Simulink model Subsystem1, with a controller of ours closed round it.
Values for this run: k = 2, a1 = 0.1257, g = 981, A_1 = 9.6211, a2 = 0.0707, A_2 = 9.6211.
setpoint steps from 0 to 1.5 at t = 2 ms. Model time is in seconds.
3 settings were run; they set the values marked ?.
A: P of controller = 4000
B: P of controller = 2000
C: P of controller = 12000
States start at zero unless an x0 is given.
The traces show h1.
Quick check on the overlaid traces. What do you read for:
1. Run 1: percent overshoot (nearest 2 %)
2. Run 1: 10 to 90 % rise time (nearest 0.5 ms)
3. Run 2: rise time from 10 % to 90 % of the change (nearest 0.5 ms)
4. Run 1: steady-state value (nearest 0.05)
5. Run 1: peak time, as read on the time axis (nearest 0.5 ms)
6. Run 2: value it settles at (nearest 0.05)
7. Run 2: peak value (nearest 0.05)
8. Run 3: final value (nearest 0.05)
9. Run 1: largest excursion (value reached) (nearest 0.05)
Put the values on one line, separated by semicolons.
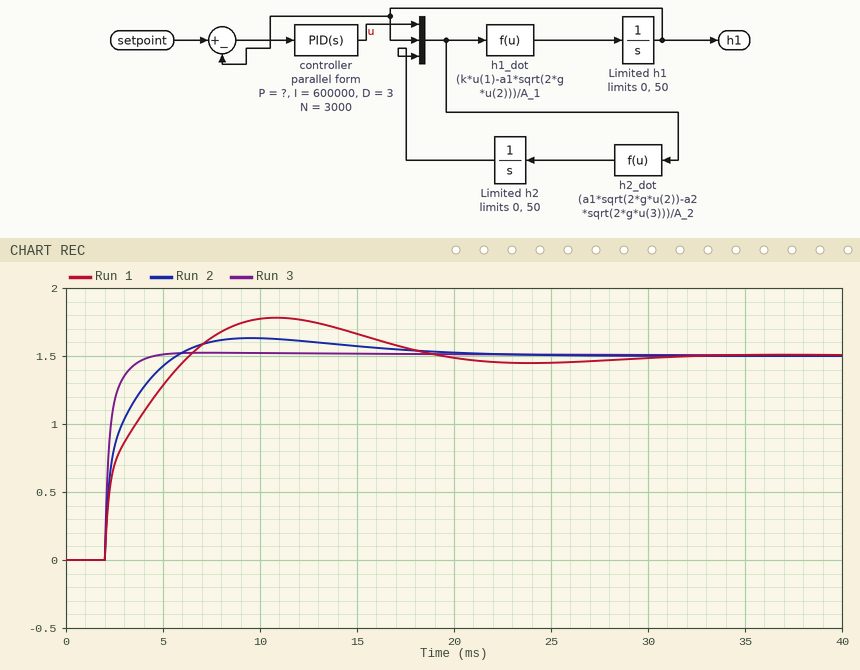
18 %; 3.5 ms; 2.5 ms; 1.50; 11.0 ms; 1.50; 1.65; 1.50; 1.80
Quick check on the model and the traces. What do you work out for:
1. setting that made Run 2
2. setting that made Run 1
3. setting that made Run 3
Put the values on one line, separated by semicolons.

A; B; C
